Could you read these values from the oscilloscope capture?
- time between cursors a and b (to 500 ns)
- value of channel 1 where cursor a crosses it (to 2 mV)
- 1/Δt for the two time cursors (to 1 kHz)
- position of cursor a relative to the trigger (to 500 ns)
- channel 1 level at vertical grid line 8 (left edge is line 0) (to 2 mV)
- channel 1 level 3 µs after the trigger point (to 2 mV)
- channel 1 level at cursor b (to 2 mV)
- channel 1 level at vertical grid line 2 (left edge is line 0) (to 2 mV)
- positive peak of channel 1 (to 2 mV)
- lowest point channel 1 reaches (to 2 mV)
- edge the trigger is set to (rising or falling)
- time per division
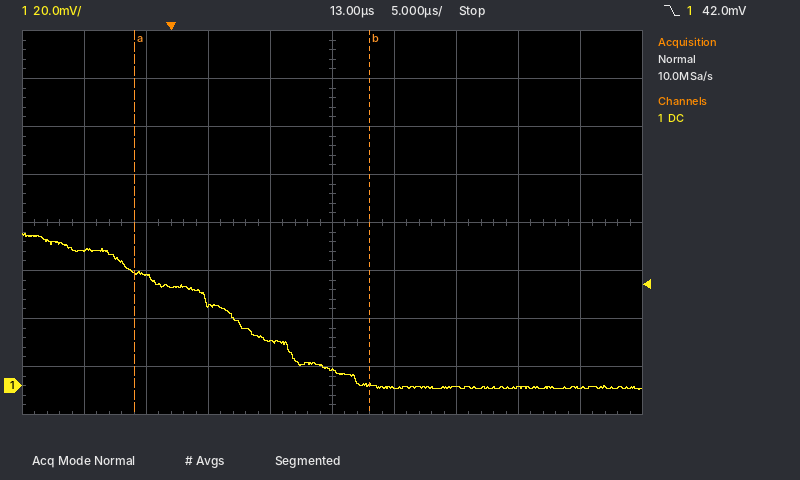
19.0 µs
48 mV
53 kHz
-3.0 µs
0 mV
34 mV
0 mV
46 mV
64 mV
-2 mV
falling
5 µs
